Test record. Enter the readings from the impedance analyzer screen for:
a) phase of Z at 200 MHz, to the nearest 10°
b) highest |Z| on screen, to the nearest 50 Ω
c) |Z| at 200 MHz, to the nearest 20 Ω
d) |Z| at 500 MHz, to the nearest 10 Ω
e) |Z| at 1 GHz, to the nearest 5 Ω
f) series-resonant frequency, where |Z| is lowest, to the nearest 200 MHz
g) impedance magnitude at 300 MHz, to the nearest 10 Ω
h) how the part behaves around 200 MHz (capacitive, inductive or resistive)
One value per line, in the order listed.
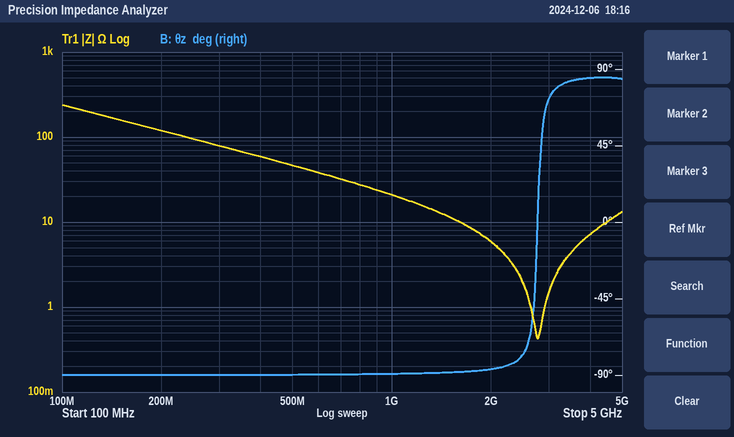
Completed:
-90°
250 Ω
120 Ω
50 Ω
20 Ω
2.8 GHz
80 Ω
capacitive
